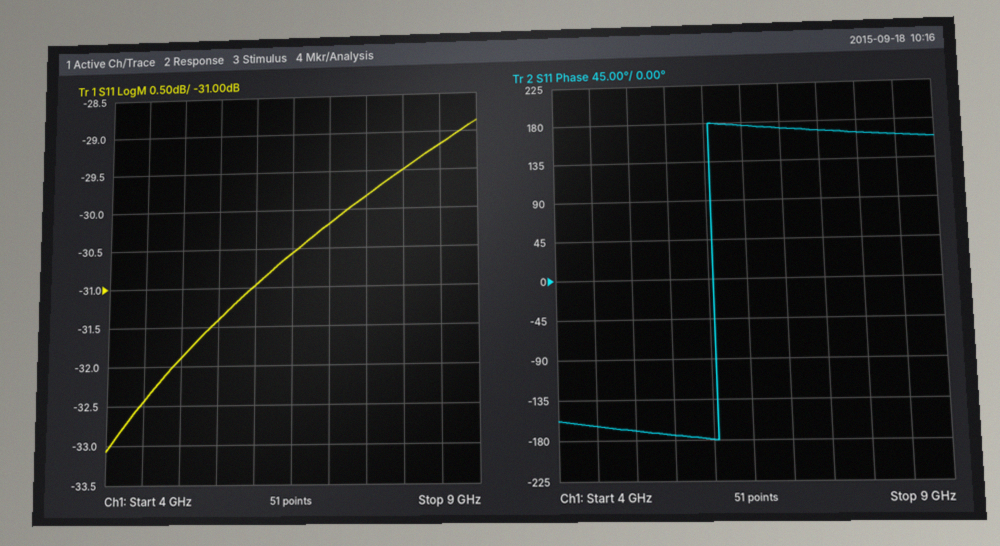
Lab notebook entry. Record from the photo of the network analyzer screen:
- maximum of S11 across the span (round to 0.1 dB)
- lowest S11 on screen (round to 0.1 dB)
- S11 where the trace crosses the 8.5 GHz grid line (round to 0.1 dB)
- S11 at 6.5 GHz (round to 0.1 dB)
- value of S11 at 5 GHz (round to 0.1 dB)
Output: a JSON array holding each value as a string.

["-28.9 dB", "-33.1 dB", "-29.2 dB", "-30.6 dB", "-31.9 dB"]
